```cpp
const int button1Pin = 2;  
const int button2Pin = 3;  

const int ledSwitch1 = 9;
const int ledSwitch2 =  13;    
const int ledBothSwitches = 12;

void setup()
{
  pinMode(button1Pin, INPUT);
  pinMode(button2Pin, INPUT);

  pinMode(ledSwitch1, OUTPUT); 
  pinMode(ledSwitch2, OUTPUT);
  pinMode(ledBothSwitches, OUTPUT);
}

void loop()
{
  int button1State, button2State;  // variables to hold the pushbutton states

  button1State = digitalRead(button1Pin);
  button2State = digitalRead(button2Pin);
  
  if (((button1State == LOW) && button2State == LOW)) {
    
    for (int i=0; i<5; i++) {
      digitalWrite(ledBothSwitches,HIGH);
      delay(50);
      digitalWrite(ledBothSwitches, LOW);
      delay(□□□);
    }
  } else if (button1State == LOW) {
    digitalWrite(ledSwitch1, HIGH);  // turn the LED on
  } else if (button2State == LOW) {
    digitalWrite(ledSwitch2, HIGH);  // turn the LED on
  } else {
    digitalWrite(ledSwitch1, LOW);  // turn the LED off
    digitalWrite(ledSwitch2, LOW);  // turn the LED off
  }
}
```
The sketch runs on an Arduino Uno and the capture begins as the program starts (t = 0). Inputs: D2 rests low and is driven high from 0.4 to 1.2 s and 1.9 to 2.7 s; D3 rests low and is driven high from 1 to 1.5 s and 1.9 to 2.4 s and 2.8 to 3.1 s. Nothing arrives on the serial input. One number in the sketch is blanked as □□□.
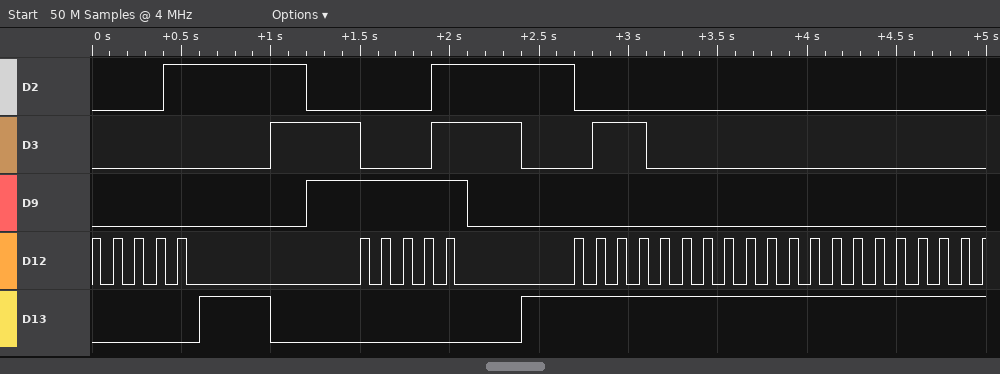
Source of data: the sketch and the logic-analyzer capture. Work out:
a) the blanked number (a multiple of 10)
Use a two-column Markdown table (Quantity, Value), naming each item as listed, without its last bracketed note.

| Quantity | Value |
|---|---|
| the blanked number | 70 |
